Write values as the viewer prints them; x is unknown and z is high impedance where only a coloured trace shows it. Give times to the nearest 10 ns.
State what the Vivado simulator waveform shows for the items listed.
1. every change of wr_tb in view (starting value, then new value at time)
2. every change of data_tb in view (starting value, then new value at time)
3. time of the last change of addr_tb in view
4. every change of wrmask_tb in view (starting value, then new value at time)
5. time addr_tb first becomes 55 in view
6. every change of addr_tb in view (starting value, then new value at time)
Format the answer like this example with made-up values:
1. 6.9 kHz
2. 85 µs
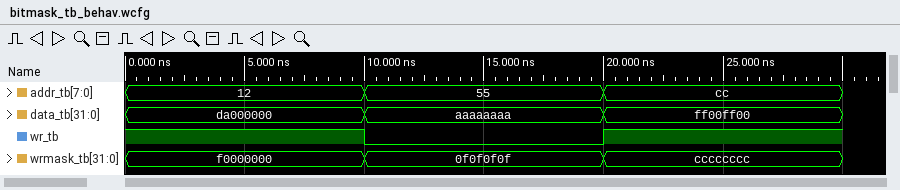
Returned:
1. 1, 0 at 10 ns, 1 at 20 ns
2. da000000, aaaaaaaa at 10 ns, ff00ff00 at 20 ns
3. 20 ns
4. f0000000, 0f0f0f0f at 10 ns, cccccccc at 20 ns
5. 10 ns
6. 12, 55 at 10 ns, cc at 20 ns
